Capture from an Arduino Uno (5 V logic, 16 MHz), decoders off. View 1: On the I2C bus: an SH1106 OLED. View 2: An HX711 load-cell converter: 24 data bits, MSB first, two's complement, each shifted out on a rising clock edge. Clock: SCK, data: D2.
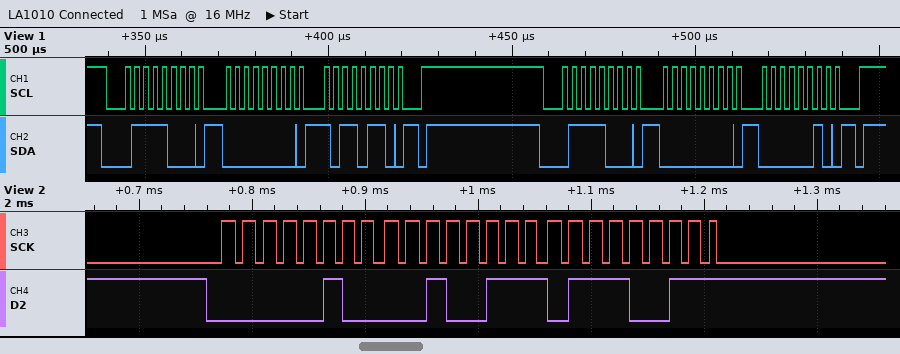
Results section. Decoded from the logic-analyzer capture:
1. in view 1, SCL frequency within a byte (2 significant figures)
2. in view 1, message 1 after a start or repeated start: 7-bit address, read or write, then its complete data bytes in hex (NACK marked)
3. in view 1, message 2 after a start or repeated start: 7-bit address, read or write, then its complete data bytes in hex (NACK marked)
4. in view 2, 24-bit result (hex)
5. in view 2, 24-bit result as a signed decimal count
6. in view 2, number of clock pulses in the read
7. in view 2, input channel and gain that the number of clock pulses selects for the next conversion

400 kHz
0x3C write: 00 B6
0x3C write: 00 02
0x042773
272243
25
channel A, gain 128
